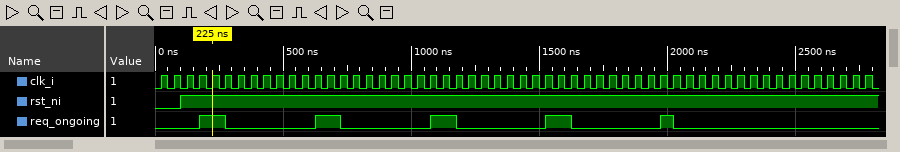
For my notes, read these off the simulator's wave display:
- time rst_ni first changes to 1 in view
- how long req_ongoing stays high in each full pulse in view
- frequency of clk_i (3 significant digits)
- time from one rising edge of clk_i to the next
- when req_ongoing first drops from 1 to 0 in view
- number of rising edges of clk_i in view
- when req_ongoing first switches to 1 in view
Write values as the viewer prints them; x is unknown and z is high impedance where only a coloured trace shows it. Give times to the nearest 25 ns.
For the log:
100 ns
100 ns, 100 ns, 100 ns, 100 ns, 50 ns
20.0 MHz
50 ns
275 ns
56
175 ns
